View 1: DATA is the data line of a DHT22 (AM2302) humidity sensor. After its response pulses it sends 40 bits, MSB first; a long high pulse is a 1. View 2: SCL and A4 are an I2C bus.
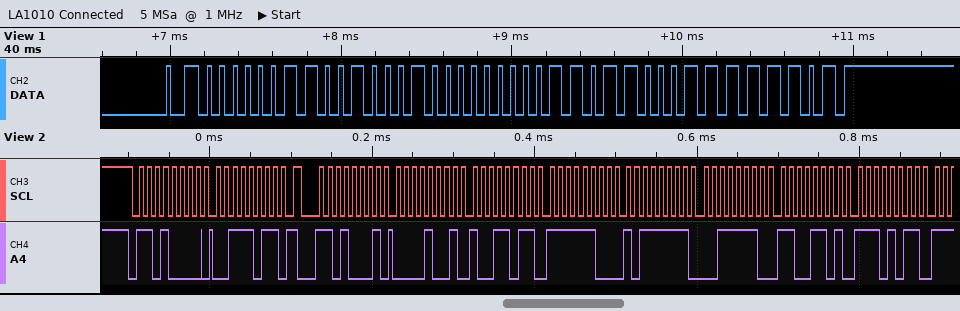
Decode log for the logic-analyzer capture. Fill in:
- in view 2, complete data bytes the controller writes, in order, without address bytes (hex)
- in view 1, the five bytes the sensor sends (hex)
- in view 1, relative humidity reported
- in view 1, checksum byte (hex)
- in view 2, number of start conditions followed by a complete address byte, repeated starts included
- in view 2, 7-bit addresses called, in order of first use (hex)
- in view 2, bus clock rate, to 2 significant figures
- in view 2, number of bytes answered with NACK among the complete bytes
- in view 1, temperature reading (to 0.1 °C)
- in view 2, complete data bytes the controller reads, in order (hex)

3B
03 22 00 D8 FD
80.2 %
0xFD
2
0x68
100 kHz
0
21.6 °C
09 9B FC BF 3E CD EB
